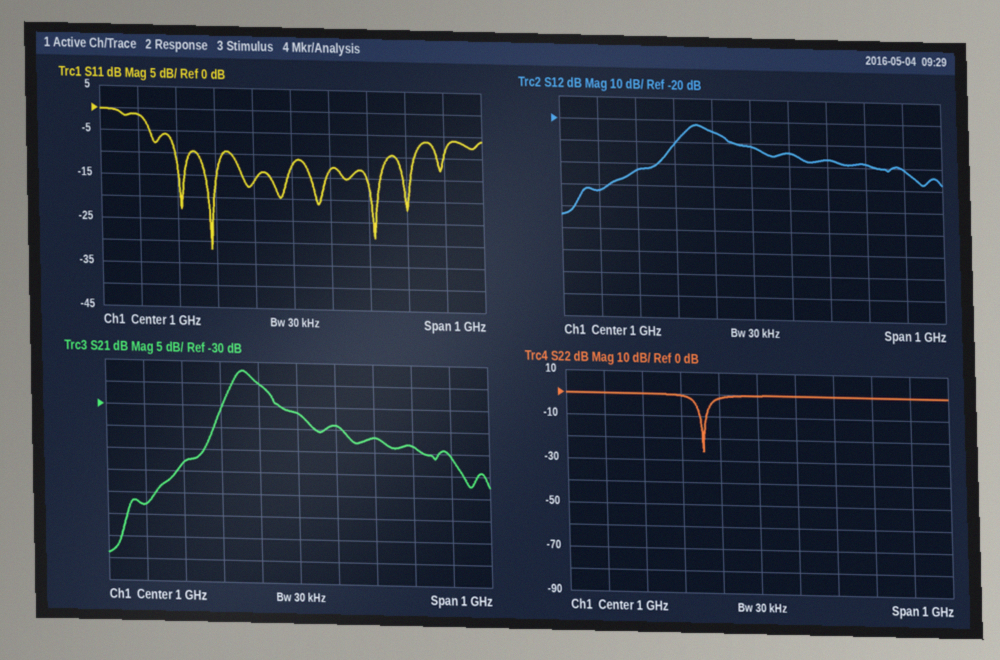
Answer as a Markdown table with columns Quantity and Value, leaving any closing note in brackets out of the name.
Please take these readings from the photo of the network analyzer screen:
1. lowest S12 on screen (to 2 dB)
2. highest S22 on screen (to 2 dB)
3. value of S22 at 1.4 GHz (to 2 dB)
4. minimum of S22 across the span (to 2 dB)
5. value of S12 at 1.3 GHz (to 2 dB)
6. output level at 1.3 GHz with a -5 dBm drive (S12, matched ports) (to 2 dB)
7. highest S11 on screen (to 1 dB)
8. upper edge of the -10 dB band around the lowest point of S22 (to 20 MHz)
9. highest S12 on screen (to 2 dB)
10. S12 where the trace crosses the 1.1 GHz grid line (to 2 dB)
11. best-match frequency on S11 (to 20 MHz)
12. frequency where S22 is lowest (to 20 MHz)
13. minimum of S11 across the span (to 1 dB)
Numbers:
| Quantity | Value |
|---|---|
| lowest S12 on screen | -64 dB |
| highest S22 on screen | 0 dB |
| value of S22 at 1.4 GHz | 0 dB |
| minimum of S22 across the span | -26 dB |
| value of S12 at 1.3 GHz | -38 dB |
| output level at 1.3 GHz with a -5 dBm drive (S12, matched ports) | -44 dBm |
| highest S11 on screen | 0 dB |
| upper edge of the -10 dB band around the lowest point of S22 | 860 MHz |
| highest S12 on screen | -22 dB |
| S12 where the trace crosses the 1.1 GHz grid line | -34 dB |
| best-match frequency on S11 | 780 MHz |
| frequency where S22 is lowest | 860 MHz |
| minimum of S11 across the span | -32 dB |
